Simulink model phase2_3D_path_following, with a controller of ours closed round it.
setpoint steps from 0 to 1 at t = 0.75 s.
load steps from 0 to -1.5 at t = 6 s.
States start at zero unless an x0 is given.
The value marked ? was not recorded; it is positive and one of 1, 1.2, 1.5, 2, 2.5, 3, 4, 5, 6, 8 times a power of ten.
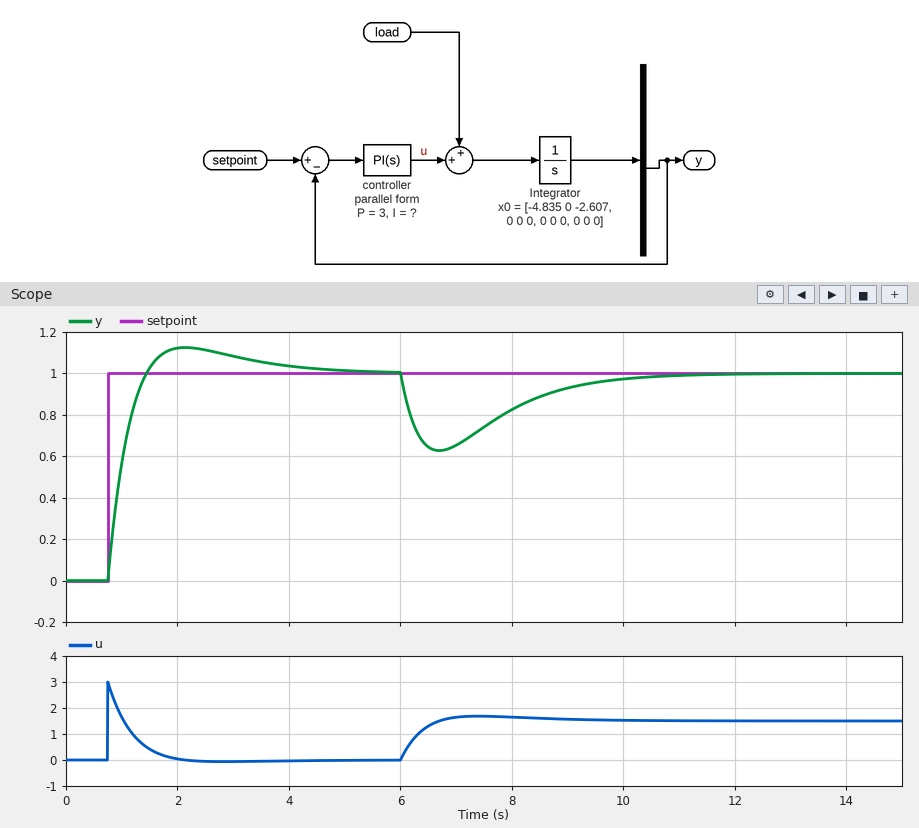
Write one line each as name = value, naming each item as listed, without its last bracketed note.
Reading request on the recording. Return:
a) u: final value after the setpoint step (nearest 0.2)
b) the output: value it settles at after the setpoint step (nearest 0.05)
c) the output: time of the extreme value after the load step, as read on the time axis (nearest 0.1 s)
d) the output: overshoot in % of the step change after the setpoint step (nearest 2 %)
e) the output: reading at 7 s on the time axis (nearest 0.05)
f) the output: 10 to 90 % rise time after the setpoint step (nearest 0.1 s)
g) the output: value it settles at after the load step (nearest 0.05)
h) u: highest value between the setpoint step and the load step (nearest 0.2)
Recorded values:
u: final value after the setpoint step = 0.0
the output: value it settles at after the setpoint step = 1.00
the output: time of the extreme value after the load step, as read on the time axis = 6.7 s
the output: overshoot in % of the step change after the setpoint step = 12 %
the output: reading at 7 s on the time axis = 0.65
the output: 10 to 90 % rise time after the setpoint step = 0.5 s
the output: value it settles at after the load step = 1.00
u: highest value between the setpoint step and the load step = 3.0
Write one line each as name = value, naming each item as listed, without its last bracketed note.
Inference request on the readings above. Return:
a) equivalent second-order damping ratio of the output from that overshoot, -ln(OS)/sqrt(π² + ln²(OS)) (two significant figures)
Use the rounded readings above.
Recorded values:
equivalent second-order damping ratio of the output from that overshoot, -ln(OS)/sqrt(π² + ln²(OS)) = 0.56
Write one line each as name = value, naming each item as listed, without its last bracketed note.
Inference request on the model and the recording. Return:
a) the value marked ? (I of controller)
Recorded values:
the value marked ? = 2
